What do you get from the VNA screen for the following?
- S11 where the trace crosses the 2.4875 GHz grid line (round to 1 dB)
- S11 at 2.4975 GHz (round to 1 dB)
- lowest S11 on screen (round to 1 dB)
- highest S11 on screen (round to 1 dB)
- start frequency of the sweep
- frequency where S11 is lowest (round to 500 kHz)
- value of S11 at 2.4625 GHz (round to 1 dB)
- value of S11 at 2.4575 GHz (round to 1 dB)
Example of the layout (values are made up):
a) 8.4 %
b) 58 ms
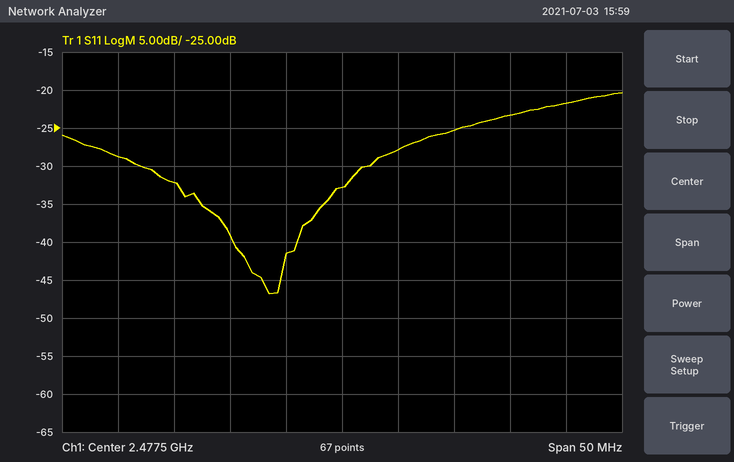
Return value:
a) -25 dB
b) -22 dB
c) -47 dB
d) -20 dB
e) 2.4525 GHz
f) 2.4710 GHz
g) -32 dB
h) -29 dB
